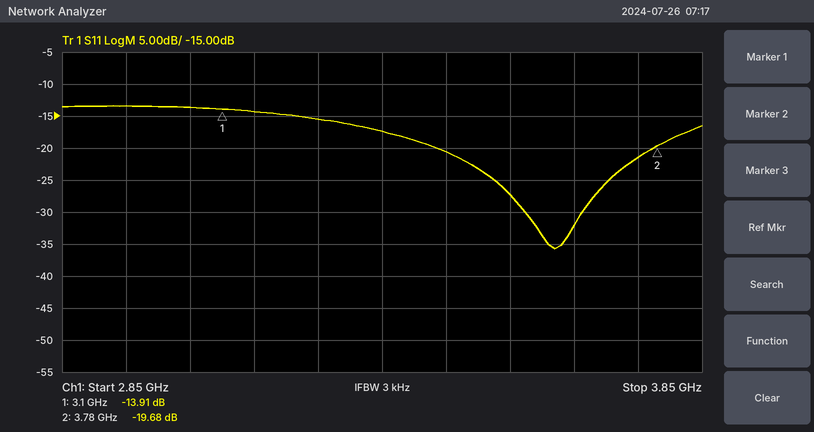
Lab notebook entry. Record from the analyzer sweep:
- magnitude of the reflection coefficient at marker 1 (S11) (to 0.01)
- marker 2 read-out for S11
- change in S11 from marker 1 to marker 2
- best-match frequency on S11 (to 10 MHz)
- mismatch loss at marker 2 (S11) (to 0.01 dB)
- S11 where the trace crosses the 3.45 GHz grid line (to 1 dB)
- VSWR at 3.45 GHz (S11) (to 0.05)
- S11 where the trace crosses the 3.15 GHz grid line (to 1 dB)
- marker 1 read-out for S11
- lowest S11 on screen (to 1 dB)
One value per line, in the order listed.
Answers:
0.20
-19.68 dB
-5.77 dB
3.62 GHz
0.05 dB
-21 dB
1.20
-14 dB
-13.91 dB
-36 dB
